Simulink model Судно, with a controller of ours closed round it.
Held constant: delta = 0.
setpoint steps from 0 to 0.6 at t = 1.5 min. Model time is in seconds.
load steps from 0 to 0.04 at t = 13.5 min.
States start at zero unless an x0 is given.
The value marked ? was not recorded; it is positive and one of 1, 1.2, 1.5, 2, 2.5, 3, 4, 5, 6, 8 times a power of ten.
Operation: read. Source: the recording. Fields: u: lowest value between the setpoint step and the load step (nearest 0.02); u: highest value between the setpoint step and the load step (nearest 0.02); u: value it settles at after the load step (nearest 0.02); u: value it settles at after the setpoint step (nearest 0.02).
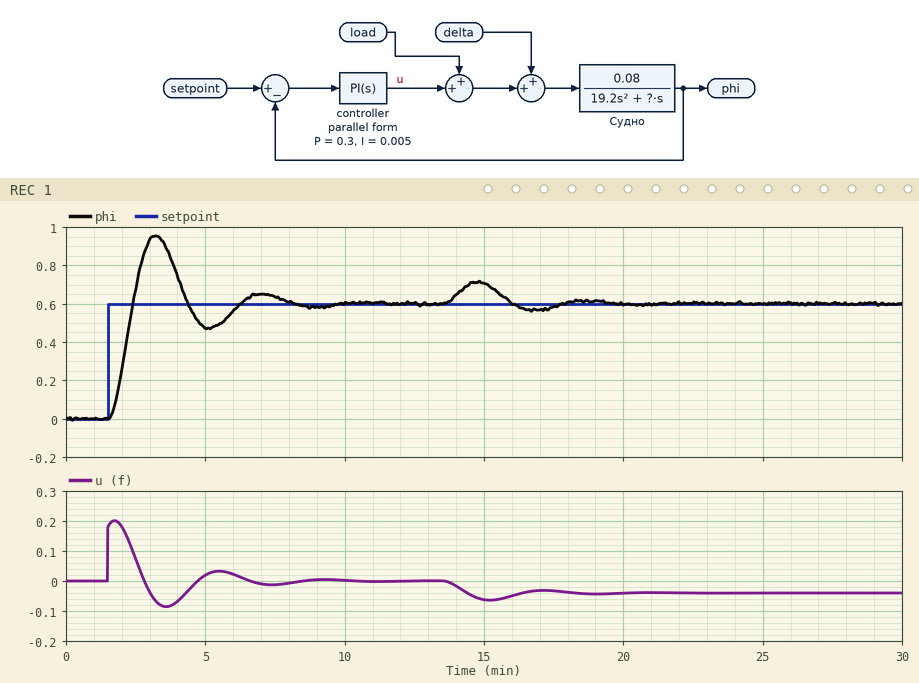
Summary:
-0.08
0.20
-0.04
0.00
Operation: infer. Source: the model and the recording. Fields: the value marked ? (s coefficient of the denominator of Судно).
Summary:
0.8
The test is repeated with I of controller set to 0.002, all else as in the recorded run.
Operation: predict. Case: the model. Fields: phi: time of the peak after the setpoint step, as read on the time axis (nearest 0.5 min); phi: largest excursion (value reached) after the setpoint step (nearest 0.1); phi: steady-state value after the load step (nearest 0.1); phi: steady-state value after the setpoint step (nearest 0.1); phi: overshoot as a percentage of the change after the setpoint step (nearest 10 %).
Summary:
3.5 min
0.8
0.6
0.6
30 %
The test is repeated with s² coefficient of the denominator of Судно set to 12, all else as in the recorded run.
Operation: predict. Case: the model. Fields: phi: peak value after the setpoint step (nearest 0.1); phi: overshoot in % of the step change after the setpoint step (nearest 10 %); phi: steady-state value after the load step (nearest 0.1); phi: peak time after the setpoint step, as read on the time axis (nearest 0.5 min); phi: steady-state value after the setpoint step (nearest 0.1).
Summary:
0.9
40 %
0.6
3.0 min
0.6
